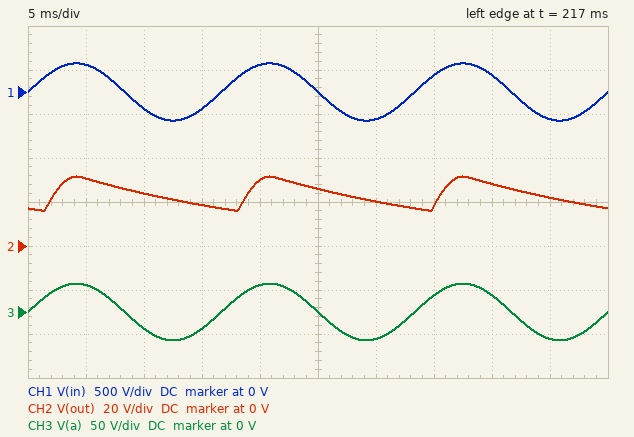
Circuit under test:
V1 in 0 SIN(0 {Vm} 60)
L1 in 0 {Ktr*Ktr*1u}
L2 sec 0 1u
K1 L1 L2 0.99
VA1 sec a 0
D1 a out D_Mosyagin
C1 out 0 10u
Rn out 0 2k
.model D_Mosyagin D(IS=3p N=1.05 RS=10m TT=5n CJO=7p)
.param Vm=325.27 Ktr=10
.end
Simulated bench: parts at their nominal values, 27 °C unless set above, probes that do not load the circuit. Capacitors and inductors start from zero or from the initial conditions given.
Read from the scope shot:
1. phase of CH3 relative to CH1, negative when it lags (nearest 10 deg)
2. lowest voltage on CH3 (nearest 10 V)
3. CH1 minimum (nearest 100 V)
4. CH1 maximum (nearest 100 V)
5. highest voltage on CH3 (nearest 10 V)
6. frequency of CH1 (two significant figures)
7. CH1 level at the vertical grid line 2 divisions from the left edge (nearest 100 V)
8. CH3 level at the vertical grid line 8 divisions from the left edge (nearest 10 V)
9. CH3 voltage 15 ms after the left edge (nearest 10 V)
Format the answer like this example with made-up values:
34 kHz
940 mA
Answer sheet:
0 deg
-30 V
-300 V
300 V
30 V
60 Hz
-200 V
20 V
-20 V
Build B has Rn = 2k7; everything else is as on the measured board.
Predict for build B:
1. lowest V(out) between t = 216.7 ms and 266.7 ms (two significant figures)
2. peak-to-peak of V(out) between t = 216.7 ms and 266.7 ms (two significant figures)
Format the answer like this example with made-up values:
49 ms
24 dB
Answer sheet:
19 V
13 V
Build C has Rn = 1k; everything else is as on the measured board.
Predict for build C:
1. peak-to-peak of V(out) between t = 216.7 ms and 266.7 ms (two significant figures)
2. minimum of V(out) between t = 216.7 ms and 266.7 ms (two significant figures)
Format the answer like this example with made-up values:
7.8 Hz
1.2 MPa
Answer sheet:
23 V
8.7 V
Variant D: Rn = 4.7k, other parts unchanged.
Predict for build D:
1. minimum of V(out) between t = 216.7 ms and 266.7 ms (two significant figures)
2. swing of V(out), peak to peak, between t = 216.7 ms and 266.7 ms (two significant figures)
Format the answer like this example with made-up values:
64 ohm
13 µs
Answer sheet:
23 V
8.4 V
